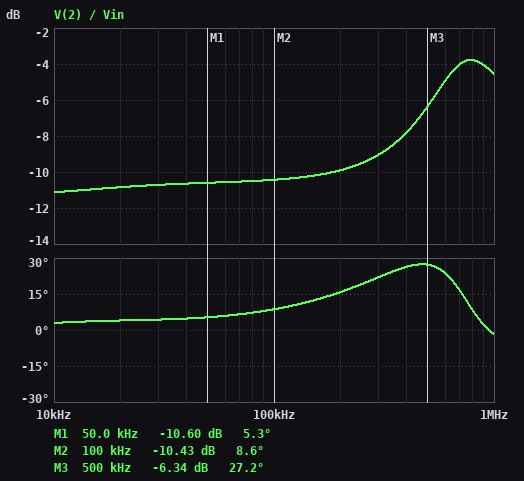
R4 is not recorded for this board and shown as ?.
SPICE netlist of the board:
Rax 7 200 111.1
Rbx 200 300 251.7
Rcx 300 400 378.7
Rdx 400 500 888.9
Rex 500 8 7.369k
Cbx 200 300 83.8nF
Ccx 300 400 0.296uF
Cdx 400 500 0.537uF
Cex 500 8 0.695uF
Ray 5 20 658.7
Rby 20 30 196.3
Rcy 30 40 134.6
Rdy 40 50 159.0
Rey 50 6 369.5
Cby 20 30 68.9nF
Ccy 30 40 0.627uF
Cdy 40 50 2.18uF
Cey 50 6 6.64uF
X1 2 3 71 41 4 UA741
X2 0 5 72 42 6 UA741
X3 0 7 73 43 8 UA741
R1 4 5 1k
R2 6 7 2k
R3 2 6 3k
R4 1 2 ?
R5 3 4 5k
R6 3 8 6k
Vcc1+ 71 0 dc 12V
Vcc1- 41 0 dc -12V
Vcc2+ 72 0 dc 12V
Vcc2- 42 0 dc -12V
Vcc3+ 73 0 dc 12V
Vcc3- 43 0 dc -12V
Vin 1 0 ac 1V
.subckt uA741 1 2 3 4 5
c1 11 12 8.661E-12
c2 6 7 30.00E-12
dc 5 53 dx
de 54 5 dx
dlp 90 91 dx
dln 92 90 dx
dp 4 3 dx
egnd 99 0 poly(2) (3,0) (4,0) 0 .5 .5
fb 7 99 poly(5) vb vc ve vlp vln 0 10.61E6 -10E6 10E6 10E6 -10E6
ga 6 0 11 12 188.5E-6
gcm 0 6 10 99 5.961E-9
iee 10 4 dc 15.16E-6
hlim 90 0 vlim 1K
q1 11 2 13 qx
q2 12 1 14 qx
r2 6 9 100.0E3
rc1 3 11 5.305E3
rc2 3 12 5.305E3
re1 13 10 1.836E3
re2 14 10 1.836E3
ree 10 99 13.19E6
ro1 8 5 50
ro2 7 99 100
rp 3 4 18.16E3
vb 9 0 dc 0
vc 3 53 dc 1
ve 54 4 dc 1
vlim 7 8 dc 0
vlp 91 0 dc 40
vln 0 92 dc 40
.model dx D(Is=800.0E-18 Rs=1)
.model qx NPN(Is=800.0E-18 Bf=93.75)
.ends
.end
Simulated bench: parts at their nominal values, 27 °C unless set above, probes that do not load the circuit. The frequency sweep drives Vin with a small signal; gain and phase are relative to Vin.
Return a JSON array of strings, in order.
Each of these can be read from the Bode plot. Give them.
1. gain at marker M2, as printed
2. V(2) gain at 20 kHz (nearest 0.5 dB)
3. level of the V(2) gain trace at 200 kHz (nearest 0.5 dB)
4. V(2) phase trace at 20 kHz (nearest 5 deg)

["-10.43 dB", "-11.0 dB", "-10.0 dB", "5 deg"]
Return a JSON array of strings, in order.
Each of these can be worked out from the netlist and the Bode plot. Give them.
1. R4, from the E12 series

["3.3 kΩ"]
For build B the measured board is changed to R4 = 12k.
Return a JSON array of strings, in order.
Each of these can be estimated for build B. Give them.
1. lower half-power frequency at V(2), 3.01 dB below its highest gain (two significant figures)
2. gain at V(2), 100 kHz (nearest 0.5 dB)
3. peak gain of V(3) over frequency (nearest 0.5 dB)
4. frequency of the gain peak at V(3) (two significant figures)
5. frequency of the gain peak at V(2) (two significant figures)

["590 kHz", "-19.5 dB", "-13.5 dB", "740 kHz", "810 kHz"]
